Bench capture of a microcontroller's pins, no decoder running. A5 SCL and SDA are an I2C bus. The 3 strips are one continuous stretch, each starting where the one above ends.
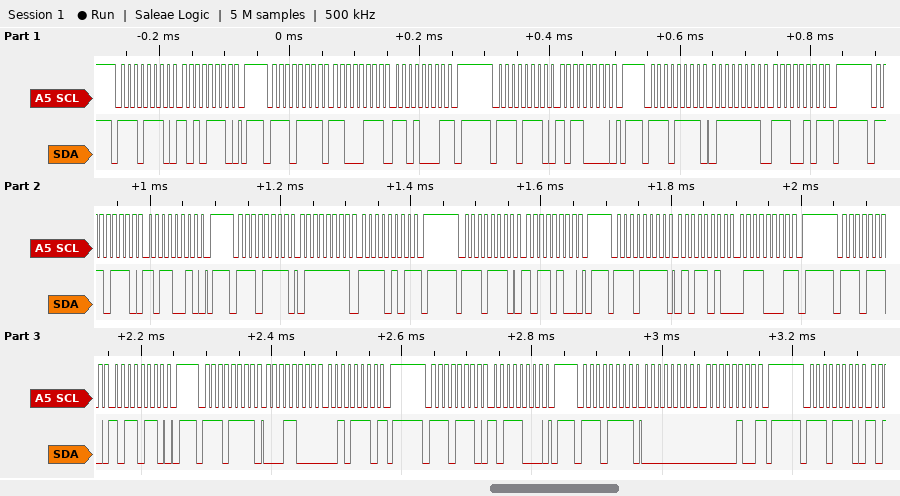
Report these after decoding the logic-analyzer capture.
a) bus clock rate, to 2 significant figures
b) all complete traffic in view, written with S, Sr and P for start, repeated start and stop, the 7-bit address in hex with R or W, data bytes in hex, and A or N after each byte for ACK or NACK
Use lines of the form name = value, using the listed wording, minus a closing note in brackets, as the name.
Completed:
bus clock rate, to 2 significant figures = 100 kHz
all complete traffic in view, written with S, Sr and P for start, repeated start and stop, the 7-bit address in hex with R or W, data bytes in hex, and A or N after each byte for ACK or NACK = S 77W A AE A P S 77R A C7 A D1 N P S 77W A B0 A P S 77R A 7F A E5 N P S 77W A B2 A P S 77R A 7F A F5 N P S 77W A B4 A P S 77R A 5A A 71 N P S 77W A B6 A P S 77R A 18 A 2E N P S 77W A B8 A P S 77R A 00 A 04 N P S 77W A
